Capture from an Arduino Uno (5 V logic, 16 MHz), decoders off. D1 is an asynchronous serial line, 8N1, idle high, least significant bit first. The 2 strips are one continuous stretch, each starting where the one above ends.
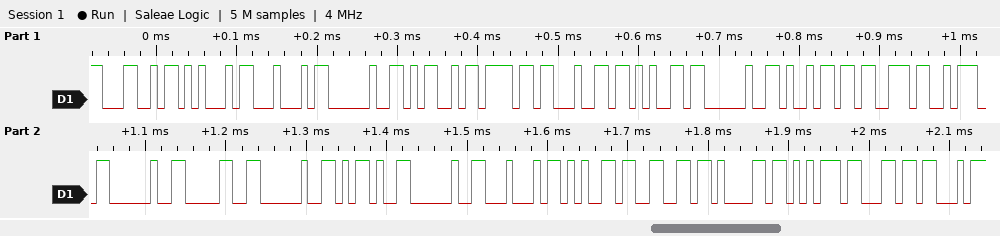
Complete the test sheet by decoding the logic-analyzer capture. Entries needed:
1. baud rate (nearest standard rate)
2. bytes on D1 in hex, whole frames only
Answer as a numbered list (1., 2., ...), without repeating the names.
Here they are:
1. 115200 baud
2. 0x4C 0x45 0x44 0x20 0x4D 0x6F 0x64 0x65 0x20 0x69 0x73 0x3A 0x20 0x30 0x20 0x2D 0x20 0x44 0x65 0x66 0x61 0x75 0x6C
